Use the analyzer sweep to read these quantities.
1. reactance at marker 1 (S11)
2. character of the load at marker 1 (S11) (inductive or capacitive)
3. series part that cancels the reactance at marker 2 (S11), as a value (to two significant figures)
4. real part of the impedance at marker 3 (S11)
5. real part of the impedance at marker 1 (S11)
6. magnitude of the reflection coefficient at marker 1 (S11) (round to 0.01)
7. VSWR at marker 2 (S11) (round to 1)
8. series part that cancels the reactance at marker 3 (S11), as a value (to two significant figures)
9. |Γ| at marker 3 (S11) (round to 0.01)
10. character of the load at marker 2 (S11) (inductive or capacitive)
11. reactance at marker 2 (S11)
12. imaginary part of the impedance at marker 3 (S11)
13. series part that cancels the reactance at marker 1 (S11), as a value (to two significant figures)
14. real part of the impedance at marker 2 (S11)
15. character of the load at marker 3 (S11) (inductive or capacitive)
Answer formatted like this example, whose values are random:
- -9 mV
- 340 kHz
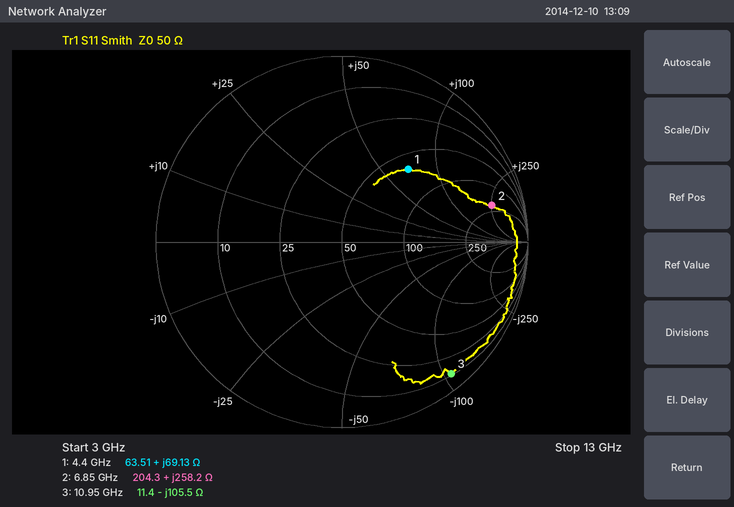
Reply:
- +69.13 Ω
- inductive
- 90 fF
- 11.4 Ω
- 63.51 Ω
- 0.53
- 11
- 1.5 nH
- 0.92
- inductive
- +258.2 Ω
- -105.5 Ω
- 520 fF
- 204.3 Ω
- capacitive
